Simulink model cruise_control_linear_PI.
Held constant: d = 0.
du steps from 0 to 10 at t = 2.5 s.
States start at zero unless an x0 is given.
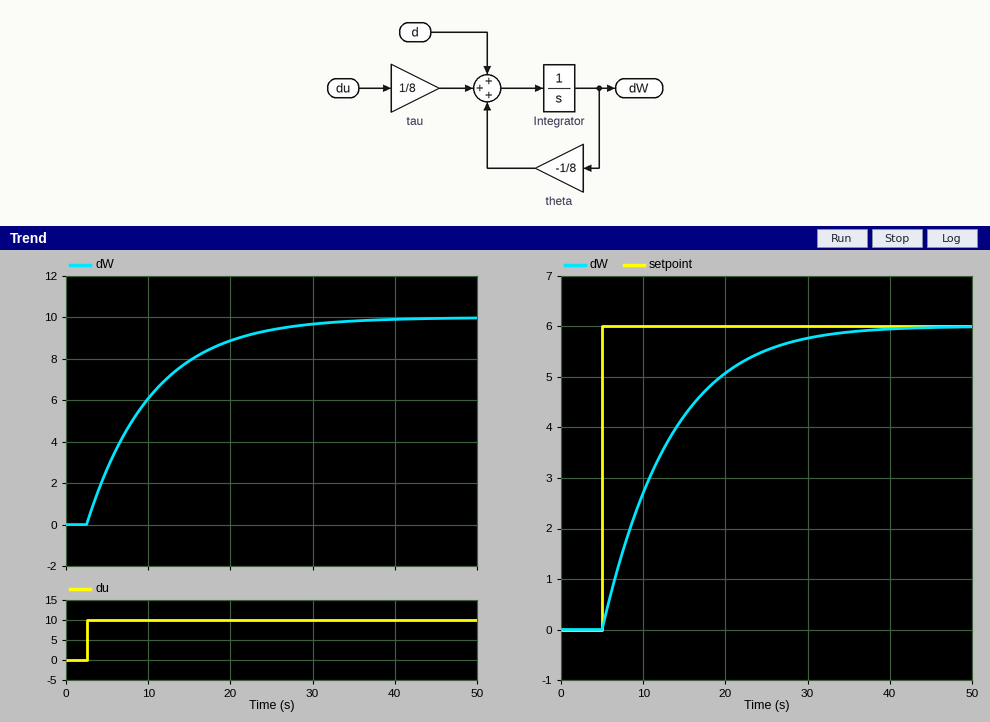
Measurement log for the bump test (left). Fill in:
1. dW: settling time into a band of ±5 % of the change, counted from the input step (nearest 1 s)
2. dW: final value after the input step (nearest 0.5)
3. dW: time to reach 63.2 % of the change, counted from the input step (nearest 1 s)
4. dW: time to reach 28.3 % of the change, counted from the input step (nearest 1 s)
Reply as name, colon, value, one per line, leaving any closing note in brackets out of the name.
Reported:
dW: settling time into a band of ±5 % of the change, counted from the input step: 24 s
dW: final value after the input step: 10.0
dW: time to reach 63.2 % of the change, counted from the input step: 8 s
dW: time to reach 28.3 % of the change, counted from the input step: 3 s
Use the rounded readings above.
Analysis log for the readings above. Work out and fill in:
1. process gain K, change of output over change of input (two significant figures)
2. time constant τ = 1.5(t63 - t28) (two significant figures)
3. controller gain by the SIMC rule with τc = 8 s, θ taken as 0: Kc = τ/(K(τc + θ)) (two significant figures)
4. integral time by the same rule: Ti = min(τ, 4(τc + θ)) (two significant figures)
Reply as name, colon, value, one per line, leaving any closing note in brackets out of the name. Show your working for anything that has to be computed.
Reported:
process gain K, change of output over change of input: (10 - 0) / 10 = 1.0
time constant τ = 1.5(t63 - t28): 1.5 × (8 - 3) = 7.5 s
controller gain by the SIMC rule with τc = 8 s, θ taken as 0: Kc = τ/(K(τc + θ)): 7.5 / (1 × (8 + 0)) = 0.94
integral time by the same rule: Ti = min(τ, 4(τc + θ)): min(7.5, 4 × (8 + 0)) = 7.5 s
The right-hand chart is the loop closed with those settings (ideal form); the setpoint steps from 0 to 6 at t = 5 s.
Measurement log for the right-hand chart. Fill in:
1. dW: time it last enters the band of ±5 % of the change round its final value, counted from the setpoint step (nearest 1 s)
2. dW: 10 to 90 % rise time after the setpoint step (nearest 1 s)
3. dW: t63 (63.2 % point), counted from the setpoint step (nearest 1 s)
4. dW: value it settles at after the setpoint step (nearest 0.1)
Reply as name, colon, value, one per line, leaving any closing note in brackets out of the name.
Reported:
dW: time it last enters the band of ±5 % of the change round its final value, counted from the setpoint step: 23 s
dW: 10 to 90 % rise time after the setpoint step: 17 s
dW: t63 (63.2 % point), counted from the setpoint step: 8 s
dW: value it settles at after the setpoint step: 6.0
